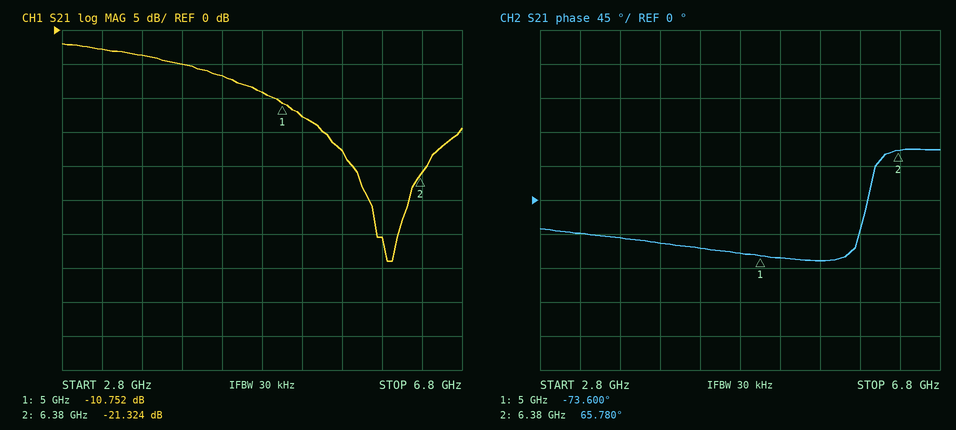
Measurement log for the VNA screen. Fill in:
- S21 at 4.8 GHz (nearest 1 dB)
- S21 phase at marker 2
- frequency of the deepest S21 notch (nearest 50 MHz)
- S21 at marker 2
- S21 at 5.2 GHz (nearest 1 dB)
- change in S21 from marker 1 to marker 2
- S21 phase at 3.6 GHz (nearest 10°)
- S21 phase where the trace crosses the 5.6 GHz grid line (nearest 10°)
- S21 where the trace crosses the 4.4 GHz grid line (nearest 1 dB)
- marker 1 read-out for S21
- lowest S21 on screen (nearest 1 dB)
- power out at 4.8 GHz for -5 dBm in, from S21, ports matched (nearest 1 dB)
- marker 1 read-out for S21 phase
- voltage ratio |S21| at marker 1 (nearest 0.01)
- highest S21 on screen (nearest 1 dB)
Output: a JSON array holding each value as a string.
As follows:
["-9 dB", "65.780°", "6.05 GHz", "-21.324 dB", "-13 dB", "-10.572 dB", "-50°", "-80°", "-7 dB", "-10.752 dB", "-34 dB", "-14 dBm", "-73.600°", "0.29", "-2 dB"]
